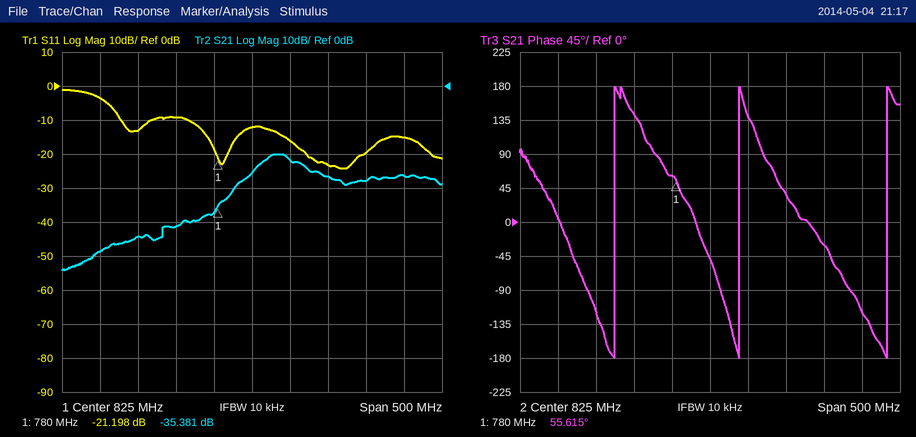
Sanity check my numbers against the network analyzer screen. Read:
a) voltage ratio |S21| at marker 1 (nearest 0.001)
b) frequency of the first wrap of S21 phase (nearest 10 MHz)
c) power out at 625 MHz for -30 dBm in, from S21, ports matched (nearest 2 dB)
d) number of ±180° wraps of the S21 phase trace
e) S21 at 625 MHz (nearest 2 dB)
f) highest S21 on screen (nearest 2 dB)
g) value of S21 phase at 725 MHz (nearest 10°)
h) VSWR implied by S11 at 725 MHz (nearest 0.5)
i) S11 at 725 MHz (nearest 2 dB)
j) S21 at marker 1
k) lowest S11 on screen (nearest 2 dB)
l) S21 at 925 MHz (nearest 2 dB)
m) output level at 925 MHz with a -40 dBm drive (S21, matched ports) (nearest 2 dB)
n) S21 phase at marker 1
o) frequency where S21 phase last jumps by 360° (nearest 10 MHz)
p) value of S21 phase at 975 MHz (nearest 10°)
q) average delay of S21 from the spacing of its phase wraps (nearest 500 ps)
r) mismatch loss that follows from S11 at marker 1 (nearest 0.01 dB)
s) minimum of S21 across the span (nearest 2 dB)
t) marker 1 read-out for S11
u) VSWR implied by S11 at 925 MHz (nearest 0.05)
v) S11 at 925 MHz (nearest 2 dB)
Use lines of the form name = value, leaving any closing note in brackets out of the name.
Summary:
voltage ratio |S21| at marker 1 = 0.017
frequency of the first wrap of S21 phase = 700 MHz
power out at 625 MHz for -30 dBm in, from S21, ports matched = -78 dBm
number of ±180° wraps of the S21 phase trace = 3
S21 at 625 MHz = -48 dB
highest S21 on screen = -20 dB
value of S21 phase at 725 MHz = 140°
VSWR implied by S11 at 725 MHz = 2.0
S11 at 725 MHz = -10 dB
S21 at marker 1 = -35.381 dB
lowest S11 on screen = -24 dB
S21 at 925 MHz = -26 dB
output level at 925 MHz with a -40 dBm drive (S21, matched ports) = -66 dBm
S21 phase at marker 1 = 55.615°
frequency where S21 phase last jumps by 360° = 1.06 GHz
value of S21 phase at 975 MHz = -30°
average delay of S21 from the spacing of its phase wraps = 5.5 ns
mismatch loss that follows from S11 at marker 1 = 0.03 dB
minimum of S21 across the span = -54 dB
marker 1 read-out for S11 = -21.198 dB
VSWR implied by S11 at 925 MHz = 1.15
S11 at 925 MHz = -24 dB
